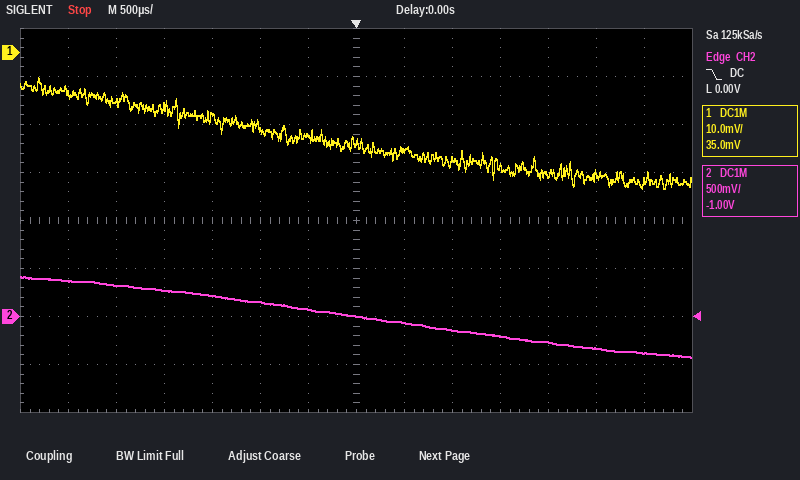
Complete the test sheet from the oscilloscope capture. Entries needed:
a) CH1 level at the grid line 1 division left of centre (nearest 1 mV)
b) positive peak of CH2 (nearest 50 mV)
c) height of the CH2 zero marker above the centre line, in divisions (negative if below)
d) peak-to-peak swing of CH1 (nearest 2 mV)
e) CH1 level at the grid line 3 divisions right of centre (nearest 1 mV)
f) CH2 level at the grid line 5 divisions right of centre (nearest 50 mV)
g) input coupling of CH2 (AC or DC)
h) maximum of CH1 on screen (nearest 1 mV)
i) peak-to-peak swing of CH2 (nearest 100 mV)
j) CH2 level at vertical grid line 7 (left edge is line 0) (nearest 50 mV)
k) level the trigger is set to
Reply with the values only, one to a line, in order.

-17 mV
400 mV
-2.0 div
24 mV
-24 mV
-350 mV
DC
-5 mV
800 mV
0 mV
0.00 V
